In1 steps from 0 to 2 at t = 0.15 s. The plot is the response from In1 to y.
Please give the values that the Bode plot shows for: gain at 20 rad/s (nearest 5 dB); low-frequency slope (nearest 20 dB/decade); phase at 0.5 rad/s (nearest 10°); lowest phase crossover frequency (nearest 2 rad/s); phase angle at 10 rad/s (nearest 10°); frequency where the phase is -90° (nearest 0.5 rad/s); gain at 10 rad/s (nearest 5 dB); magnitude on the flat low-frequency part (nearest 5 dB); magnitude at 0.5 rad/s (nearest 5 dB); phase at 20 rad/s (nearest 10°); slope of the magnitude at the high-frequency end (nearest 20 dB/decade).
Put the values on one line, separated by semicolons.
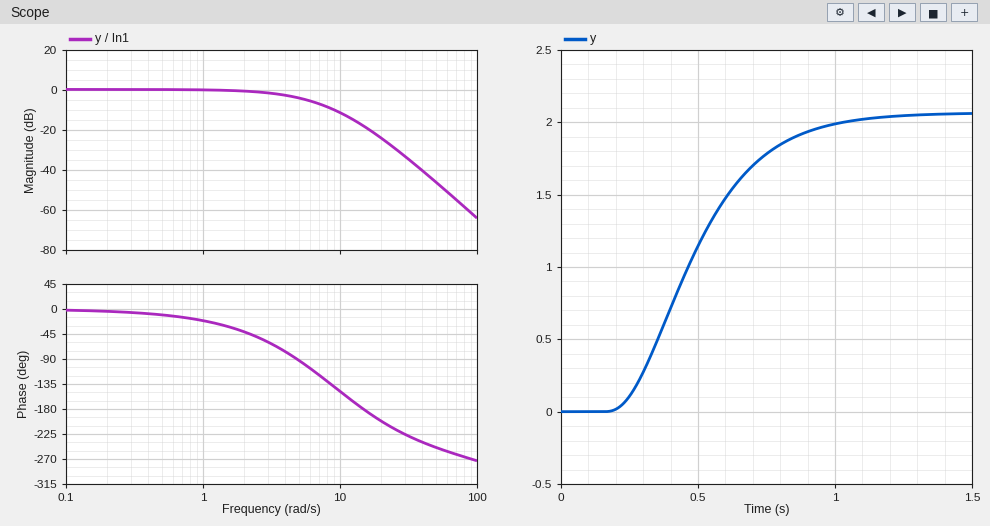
-25 dB; 0 dB/decade; -10°; 14 rad/s; -150°; 5.0 rad/s; -10 dB; 0 dB; 0 dB; -200°; -60 dB/decade
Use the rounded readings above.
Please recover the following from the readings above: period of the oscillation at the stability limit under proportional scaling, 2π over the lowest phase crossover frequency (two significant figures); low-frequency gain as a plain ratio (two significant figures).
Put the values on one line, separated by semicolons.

0.45 s; 1.0
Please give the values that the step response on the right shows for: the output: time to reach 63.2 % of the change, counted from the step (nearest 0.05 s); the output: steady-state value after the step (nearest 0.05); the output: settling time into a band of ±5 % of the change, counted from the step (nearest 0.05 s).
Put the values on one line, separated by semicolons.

0.40 s; 2.05; 0.80 s
